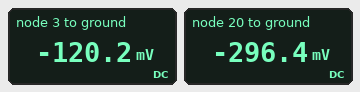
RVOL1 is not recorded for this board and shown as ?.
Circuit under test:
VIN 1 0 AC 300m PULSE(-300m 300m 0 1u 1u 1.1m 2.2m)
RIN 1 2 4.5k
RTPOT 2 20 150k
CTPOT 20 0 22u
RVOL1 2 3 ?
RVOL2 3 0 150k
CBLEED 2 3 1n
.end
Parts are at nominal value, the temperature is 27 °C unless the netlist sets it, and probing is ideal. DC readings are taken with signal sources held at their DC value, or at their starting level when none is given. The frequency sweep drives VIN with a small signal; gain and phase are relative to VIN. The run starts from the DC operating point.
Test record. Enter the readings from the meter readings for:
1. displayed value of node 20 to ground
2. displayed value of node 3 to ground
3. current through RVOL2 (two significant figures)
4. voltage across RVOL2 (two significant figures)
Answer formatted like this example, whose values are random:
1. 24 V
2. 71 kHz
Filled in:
1. -296.4 mV
2. -120.2 mV
3. 800 nA
4. 120 mV
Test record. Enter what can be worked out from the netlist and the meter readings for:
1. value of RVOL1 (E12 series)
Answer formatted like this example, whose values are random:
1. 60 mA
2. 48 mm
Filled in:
1. 220 kΩ
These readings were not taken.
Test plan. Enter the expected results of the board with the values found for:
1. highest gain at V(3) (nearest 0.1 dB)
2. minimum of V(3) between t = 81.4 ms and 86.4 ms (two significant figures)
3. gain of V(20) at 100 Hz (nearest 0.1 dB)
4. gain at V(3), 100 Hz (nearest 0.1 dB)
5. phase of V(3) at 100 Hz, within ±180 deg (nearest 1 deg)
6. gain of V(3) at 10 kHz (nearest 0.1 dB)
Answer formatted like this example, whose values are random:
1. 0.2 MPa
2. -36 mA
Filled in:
1. -0.5 dB
2. -450 mV
3. -66.7 dB
4. -8.1 dB
5. 5 deg
6. -0.6 dB
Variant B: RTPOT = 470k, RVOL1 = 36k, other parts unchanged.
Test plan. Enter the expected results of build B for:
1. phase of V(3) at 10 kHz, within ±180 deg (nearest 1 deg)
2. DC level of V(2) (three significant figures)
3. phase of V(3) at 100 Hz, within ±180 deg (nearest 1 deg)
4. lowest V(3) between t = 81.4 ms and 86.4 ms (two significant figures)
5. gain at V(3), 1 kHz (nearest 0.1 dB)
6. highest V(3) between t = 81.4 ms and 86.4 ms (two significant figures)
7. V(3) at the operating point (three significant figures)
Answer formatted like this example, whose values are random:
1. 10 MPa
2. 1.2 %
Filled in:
1. 5 deg
2. -293 mV
3. 0 deg
4. -340 mV
5. -2.1 dB
6. 340 mV
7. -236 mV
